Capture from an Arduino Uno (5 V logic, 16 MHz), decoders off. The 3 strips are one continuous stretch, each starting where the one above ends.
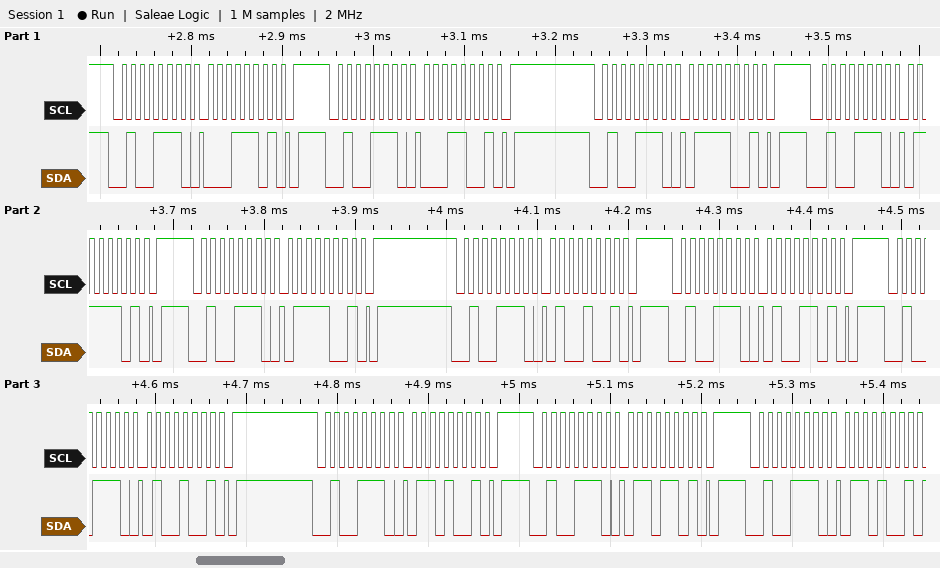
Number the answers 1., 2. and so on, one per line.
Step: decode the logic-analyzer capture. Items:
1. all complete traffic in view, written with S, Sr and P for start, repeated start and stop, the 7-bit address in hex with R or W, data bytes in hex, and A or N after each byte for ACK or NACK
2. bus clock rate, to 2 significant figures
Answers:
1. S 27W A 1D A P S 27W A 19 A P S 27W A 79 A P S 27W A 7D A P S 27W A 79 A P S 27W A 49 A P S 27W A 4D A P S 27W A 49 A P S 27W A 69 A P S 27W A 6D A P S 27W A 69 A
2. 100 kHz
